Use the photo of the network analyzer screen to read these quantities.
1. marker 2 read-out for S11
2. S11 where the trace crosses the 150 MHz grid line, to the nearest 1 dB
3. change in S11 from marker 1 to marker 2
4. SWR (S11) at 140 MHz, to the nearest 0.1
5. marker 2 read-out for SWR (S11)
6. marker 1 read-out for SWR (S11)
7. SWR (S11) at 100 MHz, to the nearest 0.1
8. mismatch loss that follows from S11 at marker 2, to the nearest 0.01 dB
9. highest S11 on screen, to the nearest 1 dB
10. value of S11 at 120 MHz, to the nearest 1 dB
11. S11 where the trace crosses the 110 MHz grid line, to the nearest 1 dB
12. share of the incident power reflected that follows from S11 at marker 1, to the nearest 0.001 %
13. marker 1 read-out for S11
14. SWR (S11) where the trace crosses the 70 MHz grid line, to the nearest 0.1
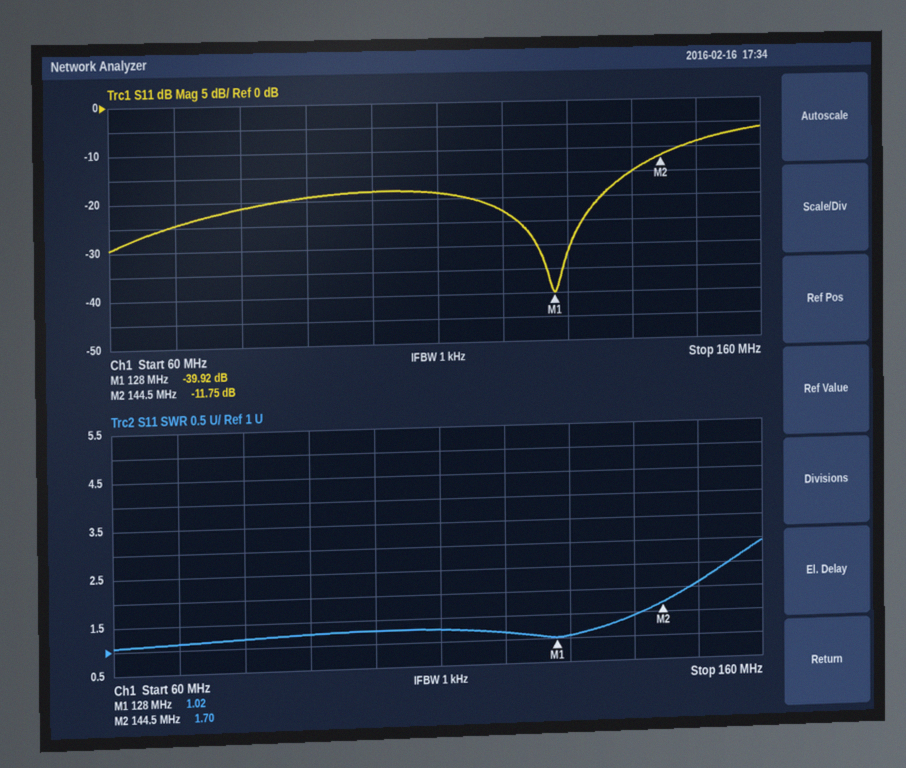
-11.75 dB
-9 dB
28.17 dB
1.4
1.70
1.02
1.3
0.30 dB
-6 dB
-23 dB
-19 dB
0.010 %
-39.92 dB
1.1
